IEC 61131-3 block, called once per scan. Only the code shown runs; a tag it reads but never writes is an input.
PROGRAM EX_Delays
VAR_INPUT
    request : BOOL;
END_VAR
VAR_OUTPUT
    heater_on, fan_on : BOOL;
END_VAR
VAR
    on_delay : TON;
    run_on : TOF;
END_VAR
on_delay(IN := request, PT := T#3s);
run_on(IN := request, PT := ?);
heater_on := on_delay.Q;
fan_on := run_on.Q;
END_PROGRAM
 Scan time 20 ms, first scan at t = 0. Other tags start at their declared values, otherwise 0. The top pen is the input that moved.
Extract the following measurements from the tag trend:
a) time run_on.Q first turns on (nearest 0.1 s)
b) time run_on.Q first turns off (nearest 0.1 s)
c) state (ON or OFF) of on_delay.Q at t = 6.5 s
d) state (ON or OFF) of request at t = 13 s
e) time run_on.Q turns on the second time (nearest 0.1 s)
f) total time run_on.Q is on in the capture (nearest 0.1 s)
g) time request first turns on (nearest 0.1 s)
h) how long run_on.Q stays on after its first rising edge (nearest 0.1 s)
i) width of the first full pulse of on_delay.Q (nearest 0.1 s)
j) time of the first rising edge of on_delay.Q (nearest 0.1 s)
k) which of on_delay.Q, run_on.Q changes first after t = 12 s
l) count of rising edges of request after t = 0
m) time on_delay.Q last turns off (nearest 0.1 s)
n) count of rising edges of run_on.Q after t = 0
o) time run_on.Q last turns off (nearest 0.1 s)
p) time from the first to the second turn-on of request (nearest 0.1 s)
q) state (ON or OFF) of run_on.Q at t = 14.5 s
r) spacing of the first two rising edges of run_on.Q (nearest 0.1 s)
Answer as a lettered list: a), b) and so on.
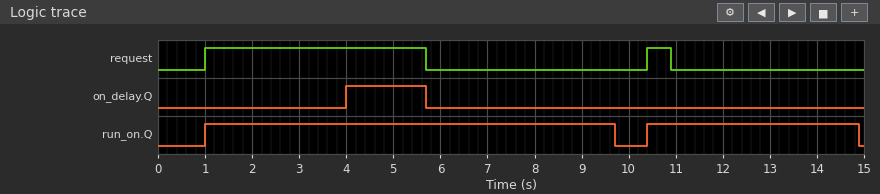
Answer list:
a) 1.0 s
b) 9.7 s
c) OFF
d) OFF
e) 10.4 s
f) 13.2 s
g) 1.0 s
h) 8.7 s
i) 1.7 s
j) 4.0 s
k) run_on.Q
l) 2
m) 5.7 s
n) 2
o) 14.9 s
p) 9.4 s
q) ON
r) 9.4 s
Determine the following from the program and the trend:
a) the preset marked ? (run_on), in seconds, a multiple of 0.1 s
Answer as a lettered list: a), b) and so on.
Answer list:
a) 4.0 s
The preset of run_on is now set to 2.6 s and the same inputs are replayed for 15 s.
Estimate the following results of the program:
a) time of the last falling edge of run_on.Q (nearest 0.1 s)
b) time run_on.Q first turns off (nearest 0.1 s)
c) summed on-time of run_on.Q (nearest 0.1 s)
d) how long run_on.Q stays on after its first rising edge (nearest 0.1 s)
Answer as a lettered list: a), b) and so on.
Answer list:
a) 13.5 s
b) 8.3 s
c) 10.4 s
d) 7.3 s
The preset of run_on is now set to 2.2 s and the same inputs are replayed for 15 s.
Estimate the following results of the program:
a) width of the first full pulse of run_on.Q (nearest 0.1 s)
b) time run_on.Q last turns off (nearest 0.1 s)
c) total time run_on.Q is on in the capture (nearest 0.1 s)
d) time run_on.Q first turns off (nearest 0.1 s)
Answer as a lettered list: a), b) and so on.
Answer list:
a) 6.9 s
b) 13.1 s
c) 9.6 s
d) 7.9 s
